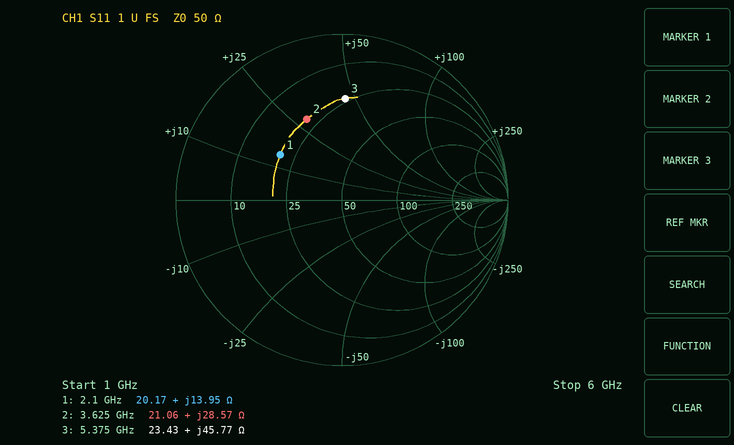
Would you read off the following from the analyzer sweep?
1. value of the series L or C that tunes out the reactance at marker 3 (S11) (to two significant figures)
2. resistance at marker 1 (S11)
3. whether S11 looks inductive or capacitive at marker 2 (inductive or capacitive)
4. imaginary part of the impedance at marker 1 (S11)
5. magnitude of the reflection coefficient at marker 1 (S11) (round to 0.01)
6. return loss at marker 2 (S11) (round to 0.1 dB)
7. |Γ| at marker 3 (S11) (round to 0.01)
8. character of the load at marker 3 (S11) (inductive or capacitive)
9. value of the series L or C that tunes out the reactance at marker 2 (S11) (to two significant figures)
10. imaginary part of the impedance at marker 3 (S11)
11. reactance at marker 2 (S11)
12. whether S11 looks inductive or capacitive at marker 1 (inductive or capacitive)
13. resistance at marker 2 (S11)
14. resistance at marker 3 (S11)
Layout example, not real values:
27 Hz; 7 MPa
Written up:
650 fF; 20.17 Ω; inductive; +13.95 Ω; 0.46; 5.5 dB; 0.61; inductive; 1.5 pF; +45.77 Ω; +28.57 Ω; inductive; 21.06 Ω; 23.43 Ω
